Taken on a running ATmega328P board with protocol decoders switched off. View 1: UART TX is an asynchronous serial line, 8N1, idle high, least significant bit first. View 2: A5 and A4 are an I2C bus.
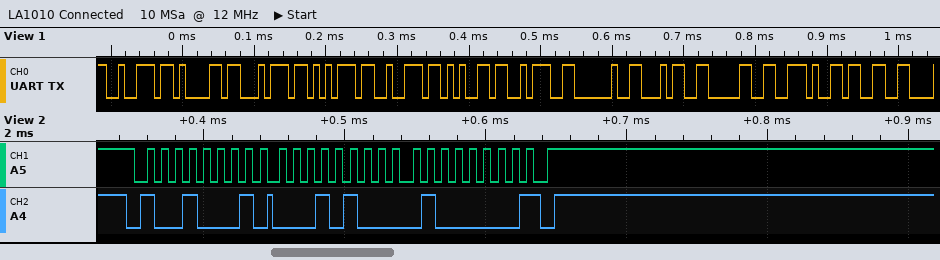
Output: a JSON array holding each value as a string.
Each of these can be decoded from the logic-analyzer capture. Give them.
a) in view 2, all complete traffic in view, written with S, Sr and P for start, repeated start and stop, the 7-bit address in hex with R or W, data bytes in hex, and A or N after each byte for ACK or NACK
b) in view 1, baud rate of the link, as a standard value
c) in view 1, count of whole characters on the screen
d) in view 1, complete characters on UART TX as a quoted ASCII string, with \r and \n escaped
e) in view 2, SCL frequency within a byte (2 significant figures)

["S 48R A 14 A 40 N P", "115200 baud", "12", "\"rature: 40.3\"", "100 kHz"]
